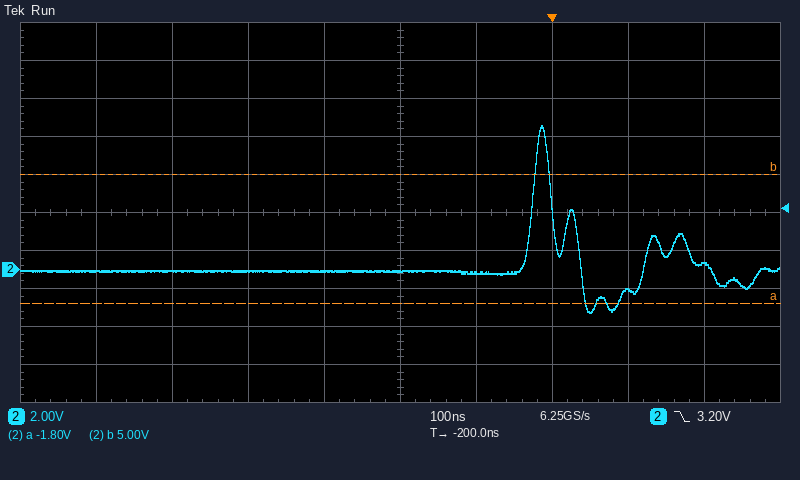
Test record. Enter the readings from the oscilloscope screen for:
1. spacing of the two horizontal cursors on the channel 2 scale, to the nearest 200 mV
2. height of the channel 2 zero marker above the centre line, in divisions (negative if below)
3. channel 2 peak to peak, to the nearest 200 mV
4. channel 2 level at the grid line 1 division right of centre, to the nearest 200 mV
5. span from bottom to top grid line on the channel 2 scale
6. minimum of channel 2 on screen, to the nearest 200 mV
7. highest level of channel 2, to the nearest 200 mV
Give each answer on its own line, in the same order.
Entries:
6.8 V
-1.5 div
9.8 V
-200 mV
20 V
-2.2 V
7.6 V
